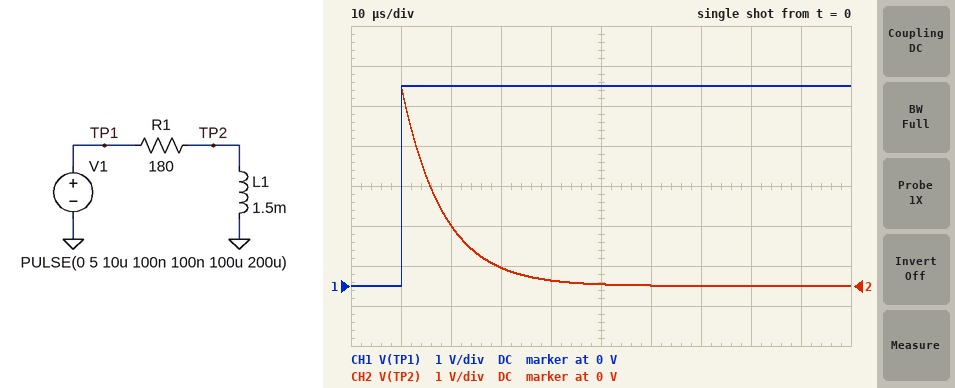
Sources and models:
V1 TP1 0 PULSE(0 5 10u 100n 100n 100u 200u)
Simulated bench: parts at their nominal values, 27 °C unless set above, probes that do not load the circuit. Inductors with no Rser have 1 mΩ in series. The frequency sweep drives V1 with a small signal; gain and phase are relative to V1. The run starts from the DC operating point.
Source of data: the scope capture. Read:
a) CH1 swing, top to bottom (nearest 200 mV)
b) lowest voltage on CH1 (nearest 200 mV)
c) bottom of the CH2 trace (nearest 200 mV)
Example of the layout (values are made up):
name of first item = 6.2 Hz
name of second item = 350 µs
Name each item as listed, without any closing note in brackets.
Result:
CH1 swing, top to bottom = 5.0 V
lowest voltage on CH1 = 0 V
bottom of the CH2 trace = 0 V
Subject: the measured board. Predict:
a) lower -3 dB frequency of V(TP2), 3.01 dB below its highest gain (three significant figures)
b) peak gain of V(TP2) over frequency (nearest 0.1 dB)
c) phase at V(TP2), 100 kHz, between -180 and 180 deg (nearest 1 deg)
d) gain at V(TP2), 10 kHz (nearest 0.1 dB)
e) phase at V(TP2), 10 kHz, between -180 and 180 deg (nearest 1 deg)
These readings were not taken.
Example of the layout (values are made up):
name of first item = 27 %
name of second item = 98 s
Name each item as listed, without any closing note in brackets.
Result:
lower -3 dB frequency of V(TP2), 3.01 dB below its highest gain = 19.1 kHz
peak gain of V(TP2) over frequency = 0 dB
phase at V(TP2), 100 kHz, between -180 and 180 deg = 11 deg
gain at V(TP2), 10 kHz = -6.7 dB
phase at V(TP2), 10 kHz, between -180 and 180 deg = 62 deg
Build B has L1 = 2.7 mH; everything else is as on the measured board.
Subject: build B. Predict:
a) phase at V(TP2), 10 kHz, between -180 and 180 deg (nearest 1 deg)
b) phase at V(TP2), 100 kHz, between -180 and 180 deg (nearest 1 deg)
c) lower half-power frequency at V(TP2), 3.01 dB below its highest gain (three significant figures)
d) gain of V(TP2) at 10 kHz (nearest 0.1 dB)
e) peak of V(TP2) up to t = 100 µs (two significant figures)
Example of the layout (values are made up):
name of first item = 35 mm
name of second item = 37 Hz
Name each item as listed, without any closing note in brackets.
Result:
phase at V(TP2), 10 kHz, between -180 and 180 deg = 47 deg
phase at V(TP2), 100 kHz, between -180 and 180 deg = 6 deg
lower half-power frequency at V(TP2), 3.01 dB below its highest gain = 10.6 kHz
gain of V(TP2) at 10 kHz = -3.3 dB
peak of V(TP2) up to t = 100 µs = 5.0 V
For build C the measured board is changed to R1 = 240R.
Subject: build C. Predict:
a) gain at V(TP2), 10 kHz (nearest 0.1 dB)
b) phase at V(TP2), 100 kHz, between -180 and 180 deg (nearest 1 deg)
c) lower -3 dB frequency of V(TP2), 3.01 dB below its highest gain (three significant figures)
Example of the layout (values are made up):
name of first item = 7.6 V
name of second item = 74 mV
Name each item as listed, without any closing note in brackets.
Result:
gain at V(TP2), 10 kHz = -8.7 dB
phase at V(TP2), 100 kHz, between -180 and 180 deg = 14 deg
lower -3 dB frequency of V(TP2), 3.01 dB below its highest gain = 25.5 kHz
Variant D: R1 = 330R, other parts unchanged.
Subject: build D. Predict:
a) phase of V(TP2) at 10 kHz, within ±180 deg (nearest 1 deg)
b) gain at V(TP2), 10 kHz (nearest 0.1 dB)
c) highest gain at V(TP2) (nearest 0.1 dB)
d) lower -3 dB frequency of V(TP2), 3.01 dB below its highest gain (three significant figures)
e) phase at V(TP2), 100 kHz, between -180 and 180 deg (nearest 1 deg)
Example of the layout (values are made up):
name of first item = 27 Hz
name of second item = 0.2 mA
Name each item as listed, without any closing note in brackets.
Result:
phase of V(TP2) at 10 kHz, within ±180 deg = 74 deg
gain at V(TP2), 10 kHz = -11.2 dB
highest gain at V(TP2) = 0 dB
lower -3 dB frequency of V(TP2), 3.01 dB below its highest gain = 35.0 kHz
phase at V(TP2), 100 kHz, between -180 and 180 deg = 19 deg
